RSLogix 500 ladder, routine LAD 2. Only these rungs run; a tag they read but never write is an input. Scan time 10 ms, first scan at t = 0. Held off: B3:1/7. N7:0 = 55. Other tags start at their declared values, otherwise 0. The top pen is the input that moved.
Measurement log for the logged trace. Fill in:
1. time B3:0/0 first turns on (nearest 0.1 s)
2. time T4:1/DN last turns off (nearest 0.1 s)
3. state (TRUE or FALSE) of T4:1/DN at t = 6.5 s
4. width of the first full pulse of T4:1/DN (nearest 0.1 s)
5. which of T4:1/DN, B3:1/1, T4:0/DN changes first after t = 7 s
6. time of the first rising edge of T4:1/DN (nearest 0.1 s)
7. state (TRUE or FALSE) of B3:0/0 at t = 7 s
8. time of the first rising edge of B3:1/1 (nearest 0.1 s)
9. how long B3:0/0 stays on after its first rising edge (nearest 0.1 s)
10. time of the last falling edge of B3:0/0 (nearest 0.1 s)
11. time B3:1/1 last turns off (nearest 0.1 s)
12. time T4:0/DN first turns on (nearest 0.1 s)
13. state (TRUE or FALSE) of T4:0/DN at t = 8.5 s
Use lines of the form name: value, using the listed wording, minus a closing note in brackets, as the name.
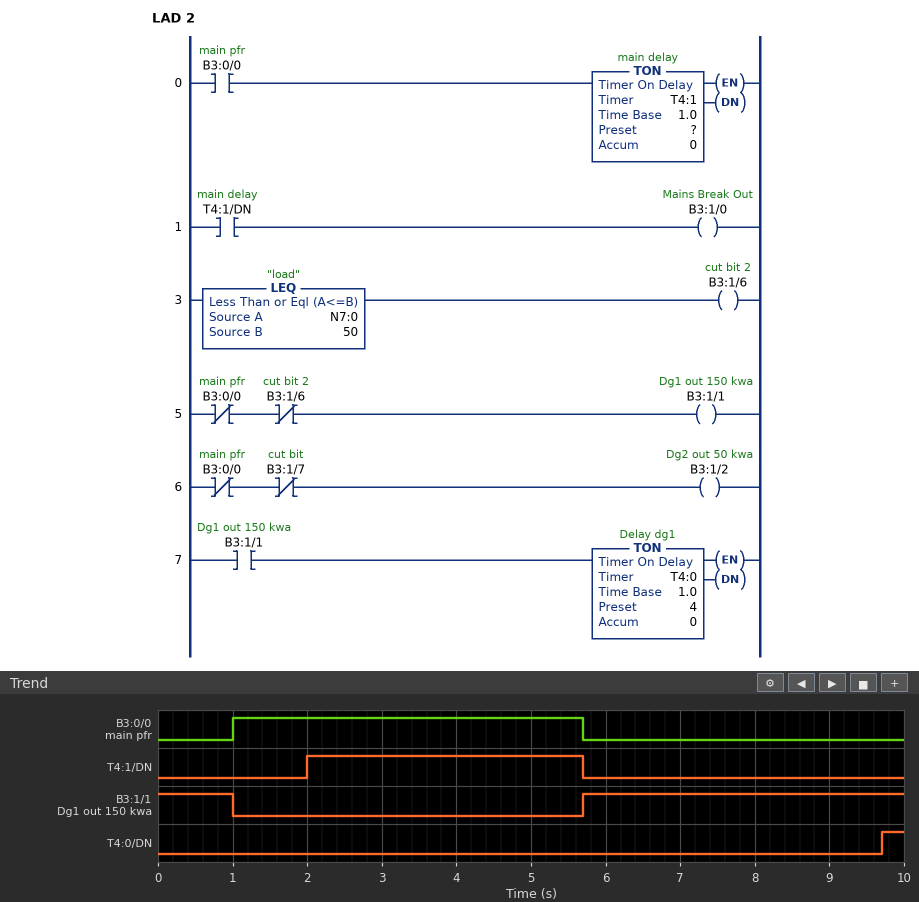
time B3:0/0 first turns on: 1.0 s
time T4:1/DN last turns off: 5.7 s
state (TRUE or FALSE) of T4:1/DN at t = 6.5 s: FALSE
width of the first full pulse of T4:1/DN: 3.7 s
which of T4:1/DN, B3:1/1, T4:0/DN changes first after t = 7 s: T4:0/DN
time of the first rising edge of T4:1/DN: 2.0 s
state (TRUE or FALSE) of B3:0/0 at t = 7 s: FALSE
time of the first rising edge of B3:1/1: 5.7 s
how long B3:0/0 stays on after its first rising edge: 4.7 s
time of the last falling edge of B3:0/0: 5.7 s
time B3:1/1 last turns off: 1.0 s
time T4:0/DN first turns on: 9.7 s
state (TRUE or FALSE) of T4:0/DN at t = 8.5 s: FALSE
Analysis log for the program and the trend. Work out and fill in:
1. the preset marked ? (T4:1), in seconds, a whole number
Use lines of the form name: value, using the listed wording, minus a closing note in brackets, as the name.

the preset marked ? (T4:1), in seconds, a whole number: 1 s
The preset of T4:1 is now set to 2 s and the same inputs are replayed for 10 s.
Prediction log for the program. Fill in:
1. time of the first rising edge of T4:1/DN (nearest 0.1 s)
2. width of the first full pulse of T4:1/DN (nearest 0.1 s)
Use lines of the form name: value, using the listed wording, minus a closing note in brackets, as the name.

time of the first rising edge of T4:1/DN: 3.0 s
width of the first full pulse of T4:1/DN: 2.7 s
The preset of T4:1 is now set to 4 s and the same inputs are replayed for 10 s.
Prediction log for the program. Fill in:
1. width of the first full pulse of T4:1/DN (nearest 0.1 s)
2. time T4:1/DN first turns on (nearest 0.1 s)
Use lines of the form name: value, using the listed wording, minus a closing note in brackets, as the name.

width of the first full pulse of T4:1/DN: 0.7 s
time T4:1/DN first turns on: 5.0 s
